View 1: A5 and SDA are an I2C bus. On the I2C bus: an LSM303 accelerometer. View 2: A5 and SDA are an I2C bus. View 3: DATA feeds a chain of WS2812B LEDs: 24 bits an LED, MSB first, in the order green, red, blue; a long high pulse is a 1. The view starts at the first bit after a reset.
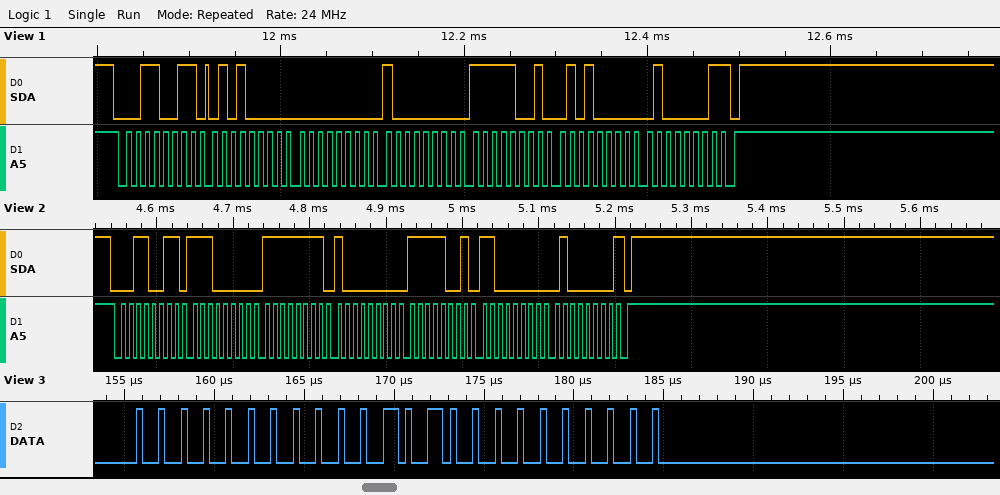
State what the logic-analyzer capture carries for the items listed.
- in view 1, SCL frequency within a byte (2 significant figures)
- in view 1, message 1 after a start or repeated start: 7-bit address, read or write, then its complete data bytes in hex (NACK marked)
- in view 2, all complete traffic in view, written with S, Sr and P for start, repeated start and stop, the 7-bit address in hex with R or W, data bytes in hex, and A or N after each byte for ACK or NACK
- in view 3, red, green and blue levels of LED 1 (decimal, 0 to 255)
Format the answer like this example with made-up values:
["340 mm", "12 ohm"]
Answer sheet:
["100 kHz", "0x19 read: 50 00 80 F9 50 41 NACK", "S 19R A E0 A FF A 80 A F9 A C0 A 40 N P", "20, 0, 0"]
